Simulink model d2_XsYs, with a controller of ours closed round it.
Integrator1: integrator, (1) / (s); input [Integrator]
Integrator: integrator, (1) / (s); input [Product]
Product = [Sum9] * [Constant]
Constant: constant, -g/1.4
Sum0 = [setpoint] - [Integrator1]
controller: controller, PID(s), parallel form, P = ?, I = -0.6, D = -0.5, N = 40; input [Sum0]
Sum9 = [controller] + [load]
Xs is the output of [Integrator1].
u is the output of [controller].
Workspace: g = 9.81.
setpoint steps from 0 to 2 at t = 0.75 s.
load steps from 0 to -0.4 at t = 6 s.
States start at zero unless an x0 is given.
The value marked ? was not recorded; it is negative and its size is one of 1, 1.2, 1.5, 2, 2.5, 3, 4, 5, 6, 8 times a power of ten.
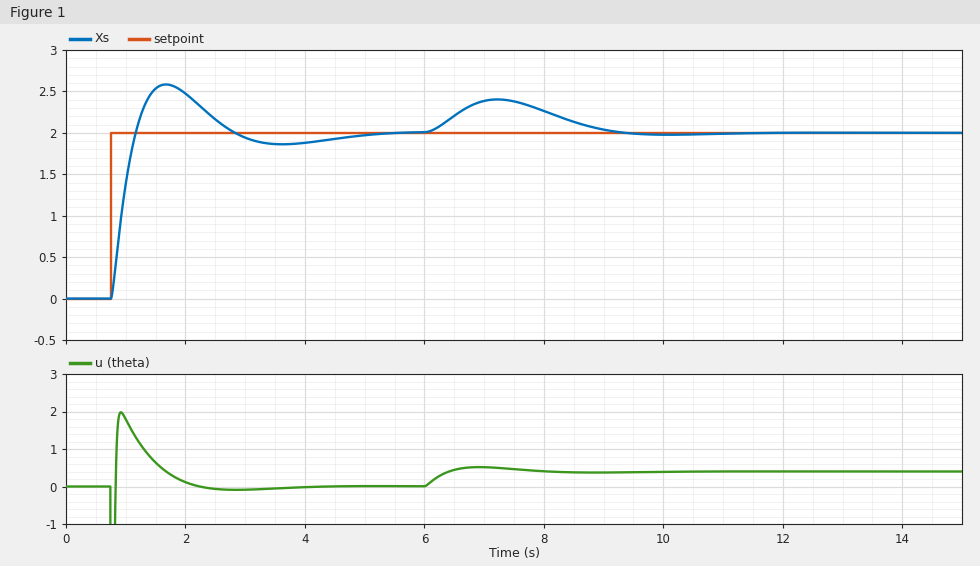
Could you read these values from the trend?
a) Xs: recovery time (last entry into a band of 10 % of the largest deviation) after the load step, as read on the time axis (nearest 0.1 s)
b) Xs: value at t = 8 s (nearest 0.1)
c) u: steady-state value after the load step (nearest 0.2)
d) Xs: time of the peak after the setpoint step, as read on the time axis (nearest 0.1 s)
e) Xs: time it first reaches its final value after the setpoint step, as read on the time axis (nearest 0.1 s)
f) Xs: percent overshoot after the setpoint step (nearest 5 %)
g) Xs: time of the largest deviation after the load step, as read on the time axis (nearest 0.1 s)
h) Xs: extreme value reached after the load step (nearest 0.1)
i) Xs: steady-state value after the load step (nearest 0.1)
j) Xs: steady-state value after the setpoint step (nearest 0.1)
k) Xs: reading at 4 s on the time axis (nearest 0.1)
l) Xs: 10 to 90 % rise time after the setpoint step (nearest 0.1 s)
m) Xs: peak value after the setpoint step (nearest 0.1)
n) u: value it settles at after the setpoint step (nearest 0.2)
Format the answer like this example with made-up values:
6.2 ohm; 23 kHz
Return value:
9.0 s; 2.3; 0.4; 1.7 s; 1.2 s; 30 %; 7.2 s; 2.4; 2.0; 2.0; 1.9; 0.3 s; 2.6; 0.0
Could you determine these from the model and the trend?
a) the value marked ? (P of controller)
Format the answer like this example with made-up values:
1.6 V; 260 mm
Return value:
-0.8
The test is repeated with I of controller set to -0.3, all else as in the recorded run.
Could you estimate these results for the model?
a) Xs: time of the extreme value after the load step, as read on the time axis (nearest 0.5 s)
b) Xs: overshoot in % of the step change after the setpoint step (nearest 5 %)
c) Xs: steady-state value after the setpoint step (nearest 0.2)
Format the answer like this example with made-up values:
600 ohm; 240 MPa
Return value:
7.5 s; 25 %; 2.0
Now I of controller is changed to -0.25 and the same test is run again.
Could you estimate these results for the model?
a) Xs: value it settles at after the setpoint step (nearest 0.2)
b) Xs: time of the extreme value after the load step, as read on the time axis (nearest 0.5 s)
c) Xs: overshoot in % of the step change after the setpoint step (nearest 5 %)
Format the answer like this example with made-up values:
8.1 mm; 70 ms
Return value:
2.0; 7.5 s; 25 %
